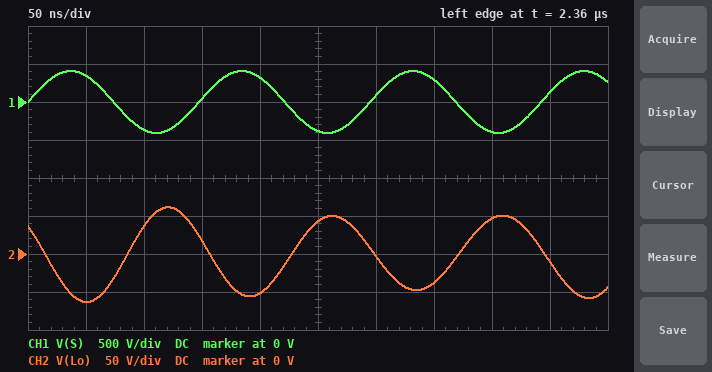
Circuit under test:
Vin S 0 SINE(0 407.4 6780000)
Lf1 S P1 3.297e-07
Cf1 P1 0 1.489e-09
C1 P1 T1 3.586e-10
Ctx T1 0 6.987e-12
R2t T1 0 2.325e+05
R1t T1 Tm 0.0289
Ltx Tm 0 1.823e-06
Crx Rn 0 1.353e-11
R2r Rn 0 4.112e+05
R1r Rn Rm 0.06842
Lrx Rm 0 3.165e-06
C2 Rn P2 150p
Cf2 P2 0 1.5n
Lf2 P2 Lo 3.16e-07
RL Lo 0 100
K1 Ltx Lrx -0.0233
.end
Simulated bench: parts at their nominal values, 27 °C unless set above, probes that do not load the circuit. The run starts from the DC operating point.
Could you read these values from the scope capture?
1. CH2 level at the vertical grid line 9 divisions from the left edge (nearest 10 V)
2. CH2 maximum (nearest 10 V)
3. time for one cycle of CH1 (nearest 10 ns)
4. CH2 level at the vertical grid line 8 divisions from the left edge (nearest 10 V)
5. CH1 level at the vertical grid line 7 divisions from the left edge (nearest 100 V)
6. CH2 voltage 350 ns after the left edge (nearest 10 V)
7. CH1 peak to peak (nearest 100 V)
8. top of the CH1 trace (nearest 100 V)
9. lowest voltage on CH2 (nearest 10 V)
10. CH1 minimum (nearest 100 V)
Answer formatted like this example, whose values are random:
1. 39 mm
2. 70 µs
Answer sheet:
1. -10 V
2. 60 V
3. 150 ns
4. 50 V
5. 300 V
6. -40 V
7. 800 V
8. 400 V
9. -60 V
10. -400 V
